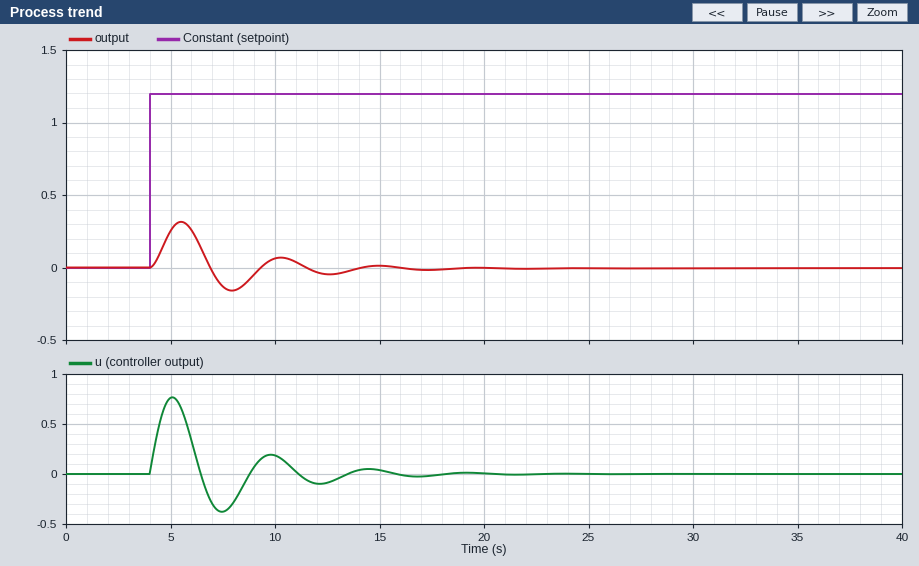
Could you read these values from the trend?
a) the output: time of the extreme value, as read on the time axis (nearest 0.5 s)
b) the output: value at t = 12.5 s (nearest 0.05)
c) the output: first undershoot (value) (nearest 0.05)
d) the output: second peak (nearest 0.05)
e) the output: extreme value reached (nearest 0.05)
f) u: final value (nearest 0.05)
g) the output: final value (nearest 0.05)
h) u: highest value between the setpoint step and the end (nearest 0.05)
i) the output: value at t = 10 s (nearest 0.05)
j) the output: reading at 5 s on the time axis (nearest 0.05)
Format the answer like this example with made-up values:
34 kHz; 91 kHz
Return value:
5.5 s; -0.05; -0.15; 0.05; 0.30; 0.00; 0.00; 0.75; 0.05; 0.25
